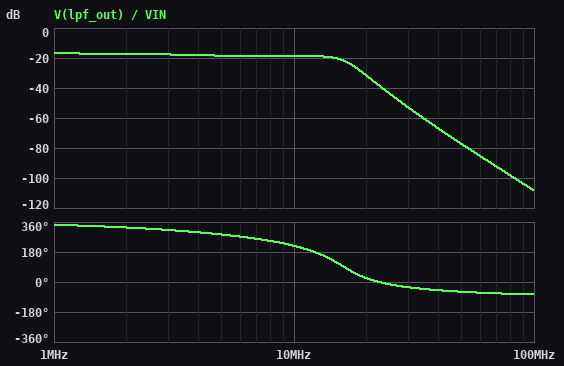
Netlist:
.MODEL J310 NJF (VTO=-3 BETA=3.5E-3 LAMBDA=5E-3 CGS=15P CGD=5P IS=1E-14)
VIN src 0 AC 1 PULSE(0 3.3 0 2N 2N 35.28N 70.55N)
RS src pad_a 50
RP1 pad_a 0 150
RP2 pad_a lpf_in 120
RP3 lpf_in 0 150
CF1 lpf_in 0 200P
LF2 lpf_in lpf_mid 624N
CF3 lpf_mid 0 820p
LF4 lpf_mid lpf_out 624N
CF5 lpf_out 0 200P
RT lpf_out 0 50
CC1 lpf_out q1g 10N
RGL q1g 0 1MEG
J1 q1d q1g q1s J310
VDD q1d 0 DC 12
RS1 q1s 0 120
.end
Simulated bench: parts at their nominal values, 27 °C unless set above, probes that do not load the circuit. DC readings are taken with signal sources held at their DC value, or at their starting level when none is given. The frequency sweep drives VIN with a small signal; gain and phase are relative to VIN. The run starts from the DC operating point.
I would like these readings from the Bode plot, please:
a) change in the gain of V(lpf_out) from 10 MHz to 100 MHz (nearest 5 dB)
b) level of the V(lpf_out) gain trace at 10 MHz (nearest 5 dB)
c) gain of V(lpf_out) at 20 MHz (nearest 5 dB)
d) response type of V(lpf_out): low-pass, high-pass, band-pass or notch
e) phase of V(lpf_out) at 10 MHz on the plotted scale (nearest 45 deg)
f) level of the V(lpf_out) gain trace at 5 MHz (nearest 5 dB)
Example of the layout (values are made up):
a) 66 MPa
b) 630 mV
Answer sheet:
a) -90 dB
b) -20 dB
c) -30 dB
d) low-pass
e) 225 deg
f) -20 dB
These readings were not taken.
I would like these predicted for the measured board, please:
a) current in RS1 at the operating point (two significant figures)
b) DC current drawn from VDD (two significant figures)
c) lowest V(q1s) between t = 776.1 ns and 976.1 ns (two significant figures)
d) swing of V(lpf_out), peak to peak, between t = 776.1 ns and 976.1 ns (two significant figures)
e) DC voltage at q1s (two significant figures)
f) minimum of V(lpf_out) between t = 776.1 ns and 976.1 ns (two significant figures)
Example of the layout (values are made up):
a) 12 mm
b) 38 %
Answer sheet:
a) 11 mA
b) 11 mA
c) 1.3 V
d) 450 mV
e) 1.3 V
f) 28 mV
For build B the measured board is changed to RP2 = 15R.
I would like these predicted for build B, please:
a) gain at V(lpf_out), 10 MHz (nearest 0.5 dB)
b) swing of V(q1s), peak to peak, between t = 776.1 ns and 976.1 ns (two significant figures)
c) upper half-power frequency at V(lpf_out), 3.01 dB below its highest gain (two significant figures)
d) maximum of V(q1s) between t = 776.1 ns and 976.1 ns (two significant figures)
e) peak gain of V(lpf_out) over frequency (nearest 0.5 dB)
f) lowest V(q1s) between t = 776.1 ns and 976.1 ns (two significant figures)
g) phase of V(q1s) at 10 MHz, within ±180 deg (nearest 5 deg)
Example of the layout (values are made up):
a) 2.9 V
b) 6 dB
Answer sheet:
a) -11.5 dB
b) 500 mV
c) 13 MHz
d) 1.9 V
e) -10.0 dB
f) 1.4 V
g) -150 deg
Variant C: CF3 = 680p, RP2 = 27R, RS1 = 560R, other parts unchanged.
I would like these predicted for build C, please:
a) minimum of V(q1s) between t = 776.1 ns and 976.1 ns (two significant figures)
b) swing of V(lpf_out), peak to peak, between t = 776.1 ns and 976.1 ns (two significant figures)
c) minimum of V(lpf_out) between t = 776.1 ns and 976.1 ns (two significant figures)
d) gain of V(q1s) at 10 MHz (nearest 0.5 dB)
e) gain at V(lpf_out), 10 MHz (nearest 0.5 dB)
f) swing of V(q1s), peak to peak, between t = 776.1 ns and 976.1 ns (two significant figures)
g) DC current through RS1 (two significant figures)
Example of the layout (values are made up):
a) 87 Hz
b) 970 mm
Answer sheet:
a) 2.0 V
b) 900 mV
c) 30 mV
d) -14.0 dB
e) -12.0 dB
f) 730 mV
g) 3.6 mA
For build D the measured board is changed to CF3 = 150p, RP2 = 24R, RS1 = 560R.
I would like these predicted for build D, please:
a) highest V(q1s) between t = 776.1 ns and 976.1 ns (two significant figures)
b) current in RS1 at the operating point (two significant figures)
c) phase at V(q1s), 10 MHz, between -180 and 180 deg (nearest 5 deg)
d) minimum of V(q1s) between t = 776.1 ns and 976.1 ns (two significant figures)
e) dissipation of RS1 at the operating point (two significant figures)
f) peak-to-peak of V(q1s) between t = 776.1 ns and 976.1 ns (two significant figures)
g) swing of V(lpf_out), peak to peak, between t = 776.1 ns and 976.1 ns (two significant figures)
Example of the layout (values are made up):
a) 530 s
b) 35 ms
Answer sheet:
a) 2.8 V
b) 3.6 mA
c) -100 deg
d) 2.0 V
e) 7.2 mW
f) 770 mV
g) 950 mV
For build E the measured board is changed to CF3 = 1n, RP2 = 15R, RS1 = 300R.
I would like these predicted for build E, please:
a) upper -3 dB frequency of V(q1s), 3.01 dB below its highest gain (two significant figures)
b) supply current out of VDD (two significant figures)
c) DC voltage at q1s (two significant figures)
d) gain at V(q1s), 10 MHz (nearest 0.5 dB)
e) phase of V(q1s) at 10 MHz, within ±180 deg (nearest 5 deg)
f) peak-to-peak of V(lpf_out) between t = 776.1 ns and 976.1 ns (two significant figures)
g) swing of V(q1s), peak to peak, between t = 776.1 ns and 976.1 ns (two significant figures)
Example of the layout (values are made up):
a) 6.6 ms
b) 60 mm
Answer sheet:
a) 11 MHz
b) 5.8 mA
c) 1.7 V
d) -15.0 dB
e) -160 deg
f) 620 mV
g) 470 mV
